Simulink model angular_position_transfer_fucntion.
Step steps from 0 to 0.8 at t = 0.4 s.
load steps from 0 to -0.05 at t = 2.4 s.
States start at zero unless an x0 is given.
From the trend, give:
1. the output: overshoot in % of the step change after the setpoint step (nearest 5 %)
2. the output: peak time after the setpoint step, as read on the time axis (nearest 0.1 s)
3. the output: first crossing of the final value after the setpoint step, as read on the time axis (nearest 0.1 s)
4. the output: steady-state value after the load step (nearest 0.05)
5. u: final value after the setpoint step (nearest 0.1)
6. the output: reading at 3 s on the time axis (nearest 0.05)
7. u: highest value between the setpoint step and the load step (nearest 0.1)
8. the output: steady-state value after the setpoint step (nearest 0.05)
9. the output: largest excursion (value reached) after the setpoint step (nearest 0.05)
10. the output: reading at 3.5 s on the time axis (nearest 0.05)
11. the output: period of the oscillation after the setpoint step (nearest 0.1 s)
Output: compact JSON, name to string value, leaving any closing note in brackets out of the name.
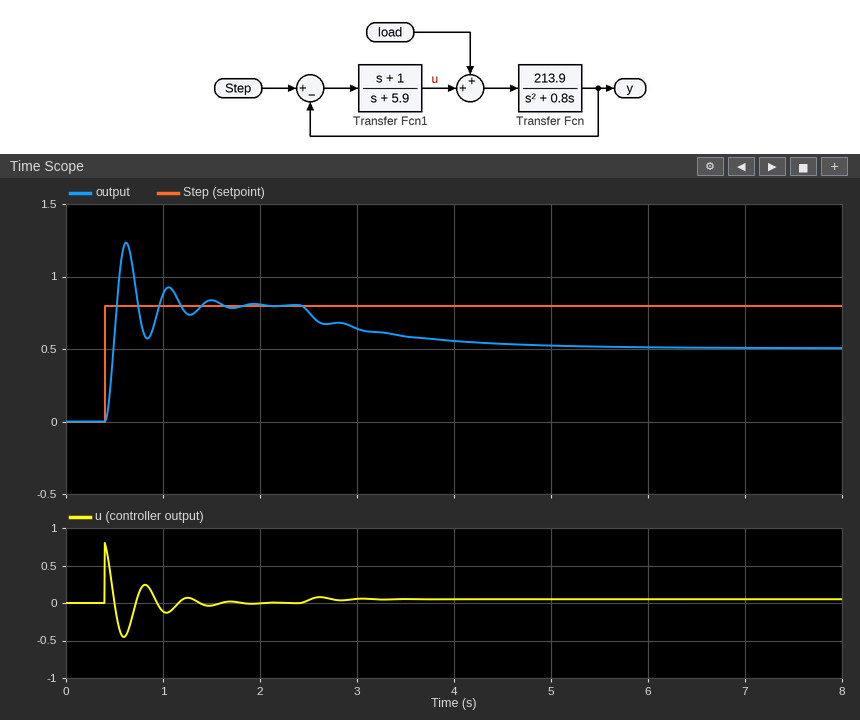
{"the output: overshoot in % of the step change after the setpoint step": "55 %", "the output: peak time after the setpoint step, as read on the time axis": "0.6 s", "the output: first crossing of the final value after the setpoint step, as read on the time axis": "0.5 s", "the output: steady-state value after the load step": "0.50", "u: final value after the setpoint step": "0.0", "the output: reading at 3 s on the time axis": "0.65", "u: highest value between the setpoint step and the load step": "0.8", "the output: steady-state value after the setpoint step": "0.80", "the output: largest excursion (value reached) after the setpoint step": "1.25", "the output: reading at 3.5 s on the time axis": "0.60", "the output: period of the oscillation after the setpoint step": "0.4 s"}
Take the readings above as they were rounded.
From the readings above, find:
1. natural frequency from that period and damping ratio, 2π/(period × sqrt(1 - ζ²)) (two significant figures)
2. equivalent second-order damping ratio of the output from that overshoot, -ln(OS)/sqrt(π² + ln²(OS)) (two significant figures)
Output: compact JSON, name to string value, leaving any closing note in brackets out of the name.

{"natural frequency from that period and damping ratio, 2π/(period × sqrt(1 - ζ²))": "16 rad/s", "equivalent second-order damping ratio of the output from that overshoot, -ln(OS)/sqrt(π² + ln²(OS))": "0.19"}
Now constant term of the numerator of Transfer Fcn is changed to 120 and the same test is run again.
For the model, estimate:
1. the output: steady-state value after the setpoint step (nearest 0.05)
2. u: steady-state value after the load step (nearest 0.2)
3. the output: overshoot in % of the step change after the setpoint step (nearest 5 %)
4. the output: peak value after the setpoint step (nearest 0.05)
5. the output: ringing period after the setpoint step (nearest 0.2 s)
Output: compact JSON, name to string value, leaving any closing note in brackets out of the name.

{"the output: steady-state value after the setpoint step": "0.80", "u: steady-state value after the load step": "0.0", "the output: overshoot in % of the step change after the setpoint step": "45 %", "the output: peak value after the setpoint step": "1.15", "the output: ringing period after the setpoint step": "0.6 s"}
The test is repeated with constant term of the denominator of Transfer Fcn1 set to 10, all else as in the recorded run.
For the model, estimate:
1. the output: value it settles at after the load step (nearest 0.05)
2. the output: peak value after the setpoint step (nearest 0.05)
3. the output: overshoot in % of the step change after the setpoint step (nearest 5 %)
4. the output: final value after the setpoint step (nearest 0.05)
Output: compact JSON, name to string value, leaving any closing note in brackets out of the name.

{"the output: value it settles at after the load step": "0.30", "the output: peak value after the setpoint step": "1.05", "the output: overshoot in % of the step change after the setpoint step": "35 %", "the output: final value after the setpoint step": "0.80"}
